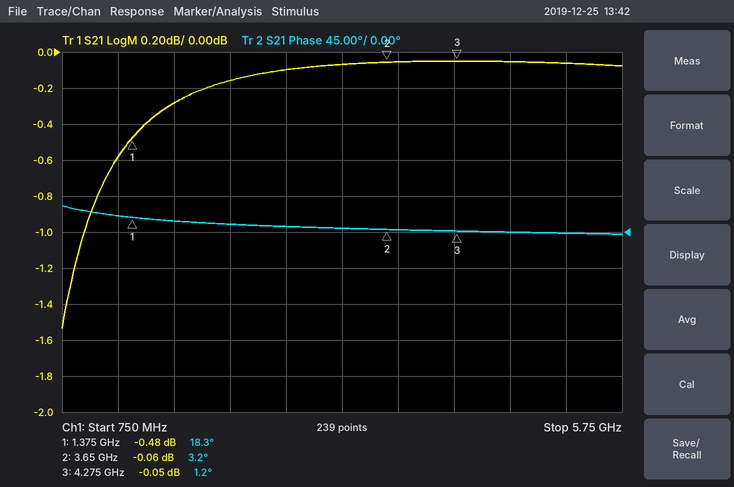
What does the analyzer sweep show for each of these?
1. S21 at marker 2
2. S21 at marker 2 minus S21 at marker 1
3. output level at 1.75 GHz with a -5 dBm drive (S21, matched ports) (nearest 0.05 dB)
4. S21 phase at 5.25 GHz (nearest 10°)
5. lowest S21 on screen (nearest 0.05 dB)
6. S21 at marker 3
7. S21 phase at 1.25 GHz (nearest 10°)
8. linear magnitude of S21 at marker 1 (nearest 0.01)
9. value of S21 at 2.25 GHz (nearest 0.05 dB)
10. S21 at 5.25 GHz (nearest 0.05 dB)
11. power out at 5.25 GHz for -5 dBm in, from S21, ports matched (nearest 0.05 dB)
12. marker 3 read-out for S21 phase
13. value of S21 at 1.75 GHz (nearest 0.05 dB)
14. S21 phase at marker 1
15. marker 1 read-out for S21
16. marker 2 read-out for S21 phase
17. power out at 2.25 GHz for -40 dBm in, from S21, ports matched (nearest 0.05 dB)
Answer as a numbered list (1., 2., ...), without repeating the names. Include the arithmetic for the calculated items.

1. -0.06 dB
2. -0.06 − (-0.48) = 0.42 dB
3. -5 dBm + (-0.30 dB) = -5.30 dBm
4. 0°
5. -1.55 dB
6. -0.05 dB
7. 20°
8. 10^(-0.48/20) ≈ 0.95
9. -0.15 dB
10. -0.05 dB
11. -5 dBm + (-0.05 dB) = -5.05 dBm
12. 1.2°
13. -0.30 dB
14. 18.3°
15. -0.48 dB
16. 3.2°
17. -40 dBm + (-0.15 dB) = -40.15 dBm
